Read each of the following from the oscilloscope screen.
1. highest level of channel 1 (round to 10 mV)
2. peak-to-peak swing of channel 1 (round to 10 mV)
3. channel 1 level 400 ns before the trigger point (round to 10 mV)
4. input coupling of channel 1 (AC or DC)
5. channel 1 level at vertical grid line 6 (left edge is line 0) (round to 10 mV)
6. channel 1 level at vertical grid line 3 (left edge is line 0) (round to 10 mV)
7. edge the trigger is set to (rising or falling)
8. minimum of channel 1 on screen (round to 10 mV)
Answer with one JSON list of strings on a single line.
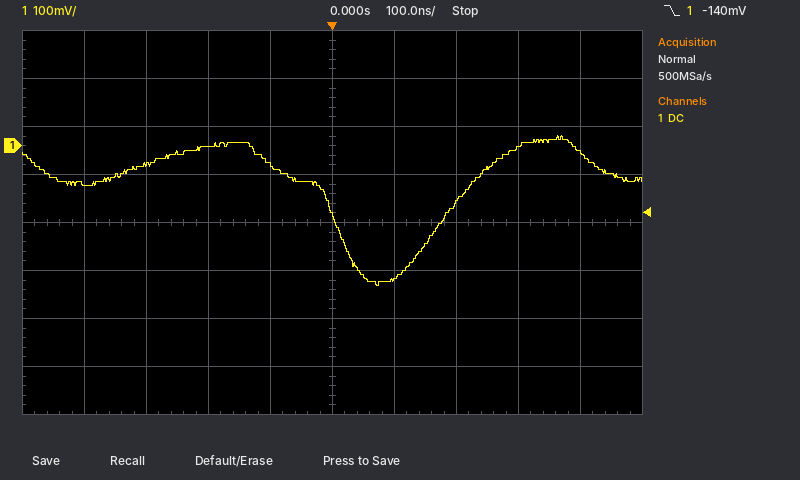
["20 mV", "310 mV", "-80 mV", "DC", "-280 mV", "0 mV", "falling", "-290 mV"]
